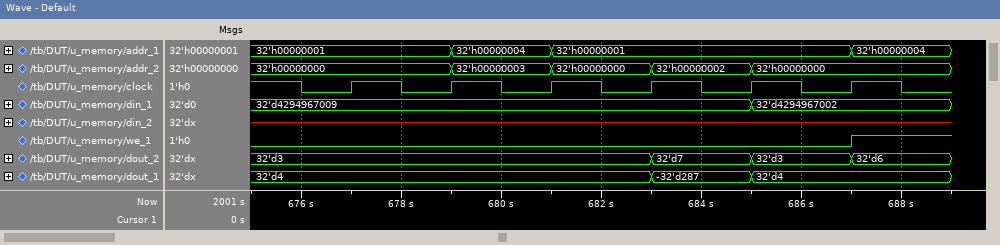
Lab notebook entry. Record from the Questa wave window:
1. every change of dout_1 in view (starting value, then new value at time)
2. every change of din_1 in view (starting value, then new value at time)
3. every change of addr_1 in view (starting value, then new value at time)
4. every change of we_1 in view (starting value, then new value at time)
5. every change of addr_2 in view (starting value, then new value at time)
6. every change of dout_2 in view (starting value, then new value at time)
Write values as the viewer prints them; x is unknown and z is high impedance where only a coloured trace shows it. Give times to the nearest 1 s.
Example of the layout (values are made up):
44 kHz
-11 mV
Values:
32'd4, -32'd287 at 683 s, 32'd4 at 685 s
32'd4294967009, 32'd4294967002 at 685 s
32'h00000001, 32'h00000004 at 679 s, 32'h00000001 at 681 s, 32'h00000004 at 687 s
0, 1 at 687 s
32'h00000000, 32'h00000003 at 679 s, 32'h00000000 at 681 s, 32'h00000002 at 683 s, 32'h00000000 at 685 s
32'd3, 32'd7 at 683 s, 32'd3 at 685 s, 32'd6 at 687 s
